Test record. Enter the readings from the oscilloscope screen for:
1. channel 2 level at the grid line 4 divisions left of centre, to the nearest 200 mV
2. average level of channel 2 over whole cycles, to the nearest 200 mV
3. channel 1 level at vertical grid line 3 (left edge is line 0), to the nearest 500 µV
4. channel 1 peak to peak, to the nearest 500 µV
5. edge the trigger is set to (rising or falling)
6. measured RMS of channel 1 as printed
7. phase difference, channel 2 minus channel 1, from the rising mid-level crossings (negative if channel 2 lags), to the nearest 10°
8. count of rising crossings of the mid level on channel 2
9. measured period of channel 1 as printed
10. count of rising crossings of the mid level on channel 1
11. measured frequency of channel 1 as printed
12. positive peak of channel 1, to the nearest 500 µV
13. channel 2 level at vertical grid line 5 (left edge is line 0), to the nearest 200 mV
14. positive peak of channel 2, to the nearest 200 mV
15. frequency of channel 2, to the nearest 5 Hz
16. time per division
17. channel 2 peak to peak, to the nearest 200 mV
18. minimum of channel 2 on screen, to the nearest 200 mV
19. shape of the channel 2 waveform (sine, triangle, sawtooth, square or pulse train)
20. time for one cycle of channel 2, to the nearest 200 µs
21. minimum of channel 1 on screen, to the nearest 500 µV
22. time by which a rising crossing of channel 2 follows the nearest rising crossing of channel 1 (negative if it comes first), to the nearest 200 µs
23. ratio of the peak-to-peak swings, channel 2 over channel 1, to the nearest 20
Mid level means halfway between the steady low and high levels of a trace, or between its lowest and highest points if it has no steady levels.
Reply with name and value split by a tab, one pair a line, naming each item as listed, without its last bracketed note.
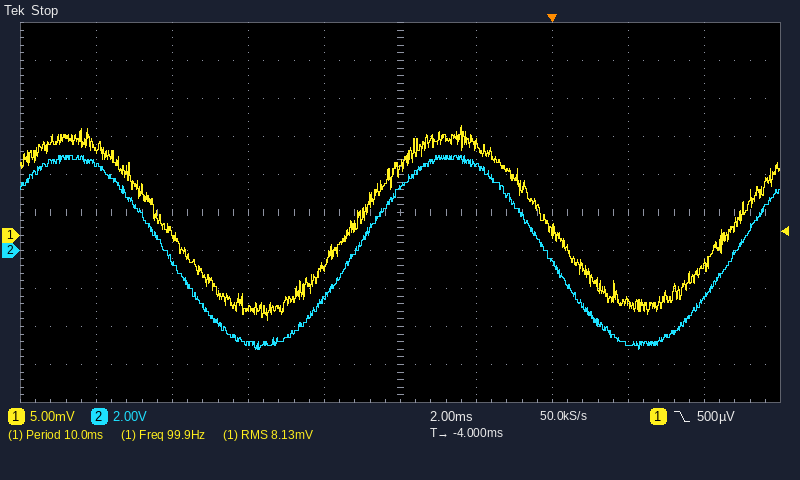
channel 2 level at the grid line 4 divisions left of centre, to the nearest 200 mV	4.6 V
average level of channel 2 over whole cycles, to the nearest 200 mV	0.0 V
channel 1 level at vertical grid line 3 (left edge is line 0), to the nearest 500 µV	-9.5 mV
channel 1 peak to peak, to the nearest 500 µV	25.5 mV
edge the trigger is set to	falling
measured RMS of channel 1 as printed	8.13 mV
phase difference, channel 2 minus channel 1, from the rising mid-level crossings (negative if channel 2 lags), to the nearest 10°	0°
count of rising crossings of the mid level on channel 2	2
measured period of channel 1 as printed	10.0 ms
count of rising crossings of the mid level on channel 1	2
measured frequency of channel 1 as printed	99.9 Hz
positive peak of channel 1, to the nearest 500 µV	14.5 mV
channel 2 level at vertical grid line 5 (left edge is line 0), to the nearest 200 mV	3.4 V
positive peak of channel 2, to the nearest 200 mV	5.0 V
frequency of channel 2, to the nearest 5 Hz	100 Hz
time per division	2 ms
channel 2 peak to peak, to the nearest 200 mV	10.2 V
minimum of channel 2 on screen, to the nearest 200 mV	-5.2 V
shape of the channel 2 waveform	sine
time for one cycle of channel 2, to the nearest 200 µs	10.0 ms
minimum of channel 1 on screen, to the nearest 500 µV	-11.0 mV
time by which a rising crossing of channel 2 follows the nearest rising crossing of channel 1 (negative if it comes first), to the nearest 200 µs	0.0 ms
ratio of the peak-to-peak swings, channel 2 over channel 1, to the nearest 20	400
